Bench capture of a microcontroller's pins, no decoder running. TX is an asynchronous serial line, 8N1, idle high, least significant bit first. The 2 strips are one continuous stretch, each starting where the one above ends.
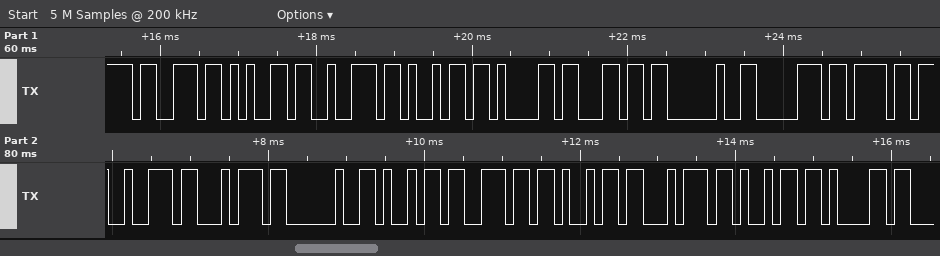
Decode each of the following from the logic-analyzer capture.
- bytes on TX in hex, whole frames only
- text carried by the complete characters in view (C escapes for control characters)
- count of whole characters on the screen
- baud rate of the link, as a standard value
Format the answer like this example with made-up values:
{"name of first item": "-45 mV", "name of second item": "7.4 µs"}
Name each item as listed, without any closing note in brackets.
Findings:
{"bytes on TX in hex, whole frames only": "73 65 72 69 61 6C 20 70 6F 72 74 20 69 6E 69 74 69 61", "text carried by the complete characters in view": "\"serial port initia\"", "count of whole characters on the screen": "18", "baud rate of the link, as a standard value": "9600 baud"}
